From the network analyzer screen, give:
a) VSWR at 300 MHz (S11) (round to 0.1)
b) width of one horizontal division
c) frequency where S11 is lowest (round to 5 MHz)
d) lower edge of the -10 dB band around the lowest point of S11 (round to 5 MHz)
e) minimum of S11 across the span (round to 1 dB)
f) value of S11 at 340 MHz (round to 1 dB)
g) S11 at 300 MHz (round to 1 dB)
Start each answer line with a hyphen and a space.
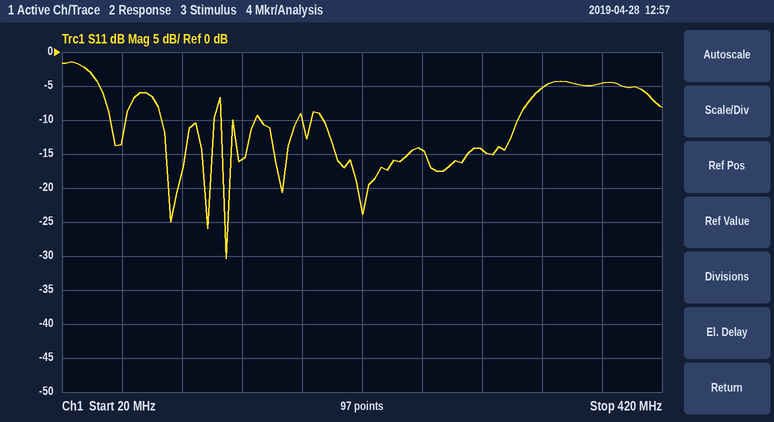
- 1.5
- 40 MHz
- 130 MHz
- 125 MHz
- -30 dB
- -5 dB
- -14 dB
